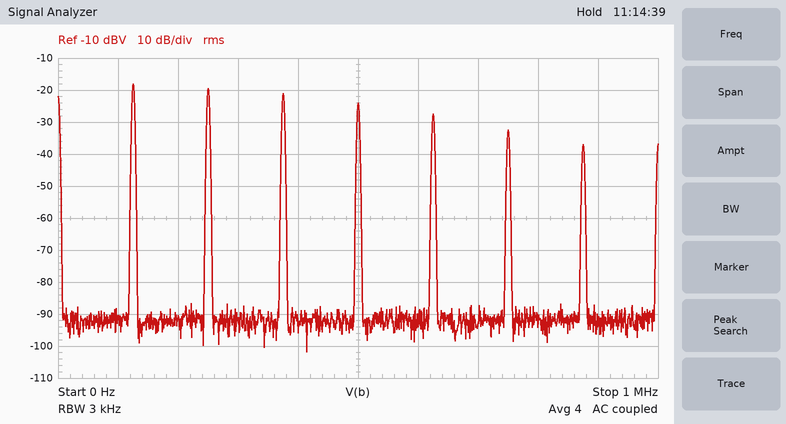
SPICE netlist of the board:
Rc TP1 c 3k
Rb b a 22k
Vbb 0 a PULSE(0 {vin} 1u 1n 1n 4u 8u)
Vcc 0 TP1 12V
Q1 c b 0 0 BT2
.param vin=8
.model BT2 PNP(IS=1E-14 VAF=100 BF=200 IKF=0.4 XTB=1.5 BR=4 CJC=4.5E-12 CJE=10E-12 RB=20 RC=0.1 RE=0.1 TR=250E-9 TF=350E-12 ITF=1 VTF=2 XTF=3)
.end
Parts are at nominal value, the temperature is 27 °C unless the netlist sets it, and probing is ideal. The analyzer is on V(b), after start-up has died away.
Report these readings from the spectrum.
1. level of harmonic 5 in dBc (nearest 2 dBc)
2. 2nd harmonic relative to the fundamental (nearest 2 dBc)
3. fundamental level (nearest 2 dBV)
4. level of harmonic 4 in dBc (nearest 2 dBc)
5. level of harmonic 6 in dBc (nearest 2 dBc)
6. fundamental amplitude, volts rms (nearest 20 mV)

-10 dBc
-2 dBc
-18 dBV
-6 dBc
-14 dBc
120 mV
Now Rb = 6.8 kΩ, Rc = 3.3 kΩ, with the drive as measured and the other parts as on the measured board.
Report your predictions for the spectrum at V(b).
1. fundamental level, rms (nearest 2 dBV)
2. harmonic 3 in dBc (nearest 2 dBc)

-16 dBV
-4 dBc
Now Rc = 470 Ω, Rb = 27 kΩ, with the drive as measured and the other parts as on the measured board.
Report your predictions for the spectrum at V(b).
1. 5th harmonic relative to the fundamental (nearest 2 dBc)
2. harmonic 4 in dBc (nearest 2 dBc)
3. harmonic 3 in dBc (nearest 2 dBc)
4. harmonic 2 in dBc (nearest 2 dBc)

-16 dBc
-14 dBc
-24 dBc
-6 dBc
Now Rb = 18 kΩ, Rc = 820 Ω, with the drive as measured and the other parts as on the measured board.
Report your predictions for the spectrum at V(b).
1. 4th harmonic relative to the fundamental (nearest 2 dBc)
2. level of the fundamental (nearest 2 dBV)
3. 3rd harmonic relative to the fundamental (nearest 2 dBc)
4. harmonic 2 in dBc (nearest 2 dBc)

-26 dBc
-12 dBV
-10 dBc
-4 dBc
